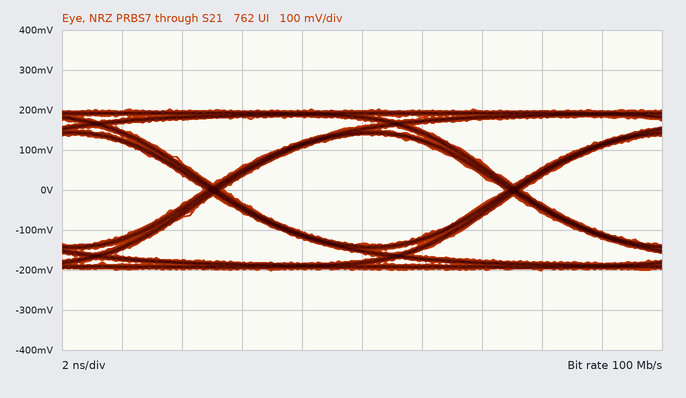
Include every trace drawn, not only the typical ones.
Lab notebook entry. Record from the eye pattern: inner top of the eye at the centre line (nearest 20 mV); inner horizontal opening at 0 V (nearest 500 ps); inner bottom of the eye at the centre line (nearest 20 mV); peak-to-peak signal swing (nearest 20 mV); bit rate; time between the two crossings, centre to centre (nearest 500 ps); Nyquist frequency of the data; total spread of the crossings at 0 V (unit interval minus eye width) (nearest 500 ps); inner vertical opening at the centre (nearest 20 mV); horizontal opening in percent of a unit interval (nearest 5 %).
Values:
140 mV
9.5 ns
-140 mV
400 mV
100 Mb/s
10.0 ns
50 MHz
500 ps
280 mV
95 %
